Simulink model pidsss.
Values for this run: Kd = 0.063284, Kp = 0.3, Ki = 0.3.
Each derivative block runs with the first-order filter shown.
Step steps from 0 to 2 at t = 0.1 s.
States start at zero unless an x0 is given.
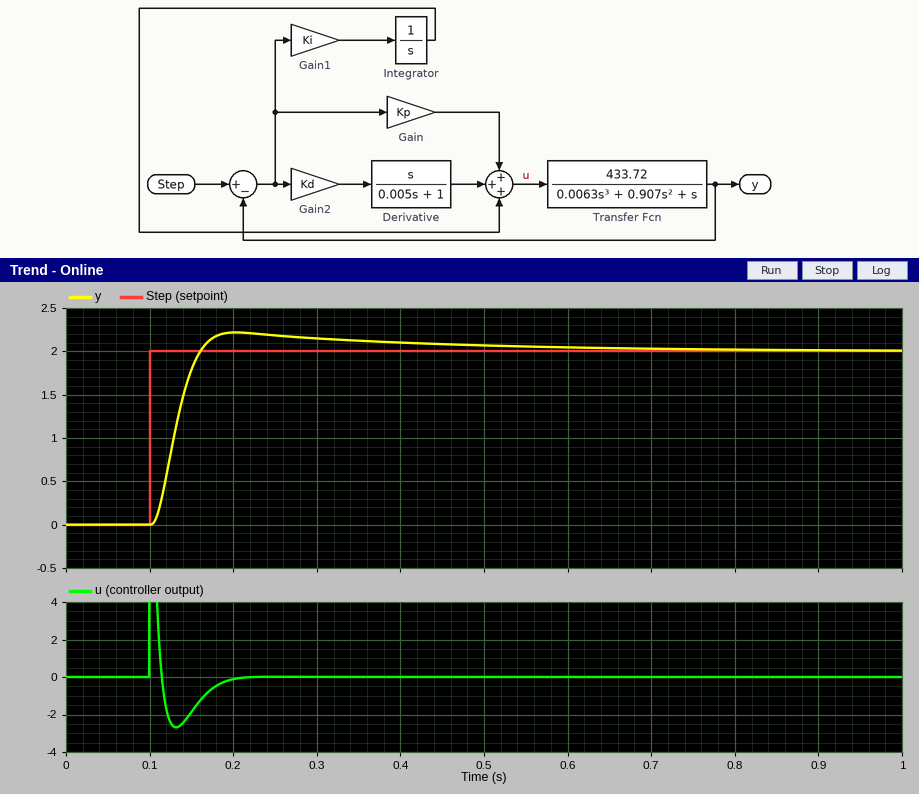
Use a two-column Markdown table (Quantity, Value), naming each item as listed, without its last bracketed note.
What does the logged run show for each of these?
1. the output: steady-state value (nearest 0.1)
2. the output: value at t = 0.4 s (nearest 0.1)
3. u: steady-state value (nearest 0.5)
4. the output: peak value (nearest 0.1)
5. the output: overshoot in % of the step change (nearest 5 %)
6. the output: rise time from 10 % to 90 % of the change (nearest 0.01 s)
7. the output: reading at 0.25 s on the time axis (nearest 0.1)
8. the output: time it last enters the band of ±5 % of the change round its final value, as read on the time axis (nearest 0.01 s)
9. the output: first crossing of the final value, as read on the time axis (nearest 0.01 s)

| Quantity | Value |
|---|---|
| the output: steady-state value | 2.0 |
| the output: value at t = 0.4 s | 2.1 |
| u: steady-state value | 0.0 |
| the output: peak value | 2.2 |
| the output: overshoot in % of the step change | 10 % |
| the output: rise time from 10 % to 90 % of the change | 0.04 s |
| the output: reading at 0.25 s on the time axis | 2.2 |
| the output: time it last enters the band of ±5 % of the change round its final value, as read on the time axis | 0.40 s |
| the output: first crossing of the final value, as read on the time axis | 0.16 s |
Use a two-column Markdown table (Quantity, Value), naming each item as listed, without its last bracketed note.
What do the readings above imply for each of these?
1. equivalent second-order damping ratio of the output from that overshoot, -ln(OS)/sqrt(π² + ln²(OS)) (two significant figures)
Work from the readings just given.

| Quantity | Value |
|---|---|
| equivalent second-order damping ratio of the output from that overshoot, -ln(OS)/sqrt(π² + ln²(OS)) | 0.59 |
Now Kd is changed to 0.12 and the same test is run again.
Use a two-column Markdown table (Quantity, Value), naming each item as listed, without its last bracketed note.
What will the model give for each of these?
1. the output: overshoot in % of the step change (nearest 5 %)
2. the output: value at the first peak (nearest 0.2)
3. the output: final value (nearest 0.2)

| Quantity | Value |
|---|---|
| the output: overshoot in % of the step change | 15 % |
| the output: value at the first peak | 2.4 |
| the output: final value | 2.0 |
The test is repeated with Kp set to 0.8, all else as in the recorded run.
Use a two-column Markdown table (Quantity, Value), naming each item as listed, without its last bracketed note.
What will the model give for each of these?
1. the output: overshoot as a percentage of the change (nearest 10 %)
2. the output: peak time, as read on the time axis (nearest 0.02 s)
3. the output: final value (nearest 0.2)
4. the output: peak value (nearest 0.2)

| Quantity | Value |
|---|---|
| the output: overshoot as a percentage of the change | 30 % |
| the output: peak time, as read on the time axis | 0.18 s |
| the output: final value | 2.0 |
| the output: peak value | 2.6 |
